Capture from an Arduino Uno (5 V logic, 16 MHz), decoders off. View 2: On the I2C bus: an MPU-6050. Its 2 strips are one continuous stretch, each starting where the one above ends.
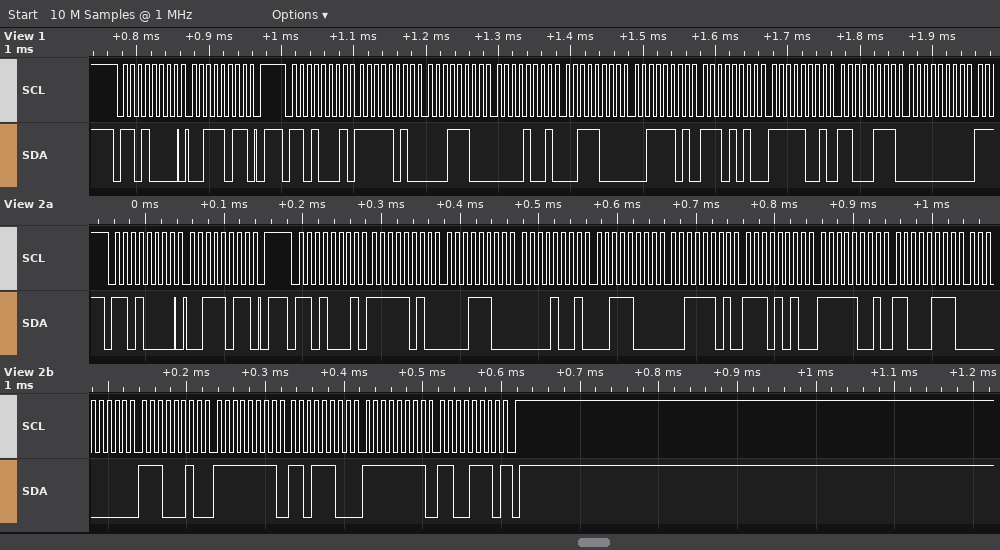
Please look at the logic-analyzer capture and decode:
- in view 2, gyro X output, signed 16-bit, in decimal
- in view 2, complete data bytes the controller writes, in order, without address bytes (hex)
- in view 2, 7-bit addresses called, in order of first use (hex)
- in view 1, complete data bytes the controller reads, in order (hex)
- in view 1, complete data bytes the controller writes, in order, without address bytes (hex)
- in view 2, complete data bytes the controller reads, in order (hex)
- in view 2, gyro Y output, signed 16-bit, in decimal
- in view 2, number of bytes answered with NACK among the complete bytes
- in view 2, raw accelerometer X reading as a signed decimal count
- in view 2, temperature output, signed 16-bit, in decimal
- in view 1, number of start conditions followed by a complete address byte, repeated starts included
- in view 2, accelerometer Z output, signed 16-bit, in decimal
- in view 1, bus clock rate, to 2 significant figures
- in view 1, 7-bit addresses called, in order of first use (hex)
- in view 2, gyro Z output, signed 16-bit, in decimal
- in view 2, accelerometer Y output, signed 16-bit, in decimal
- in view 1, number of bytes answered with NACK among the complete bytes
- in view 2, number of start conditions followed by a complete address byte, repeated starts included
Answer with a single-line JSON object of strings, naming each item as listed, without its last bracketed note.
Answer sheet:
{"in view 2, gyro X output, signed 16-bit, in decimal": "226", "in view 2, complete data bytes the controller writes, in order, without address bytes": "3B", "in view 2, 7-bit addresses called, in order of first use": "0x68", "in view 1, complete data bytes the controller reads, in order": "FA 1C 09 38 3D EA F9 C7 00", "in view 1, complete data bytes the controller writes, in order, without address bytes": "3B", "in view 2, complete data bytes the controller reads, in order": "FA 1C 09 38 3D EA F9 C7 00 E2 FF DC FF CE", "in view 2, gyro Y output, signed 16-bit, in decimal": "-36", "in view 2, number of bytes answered with NACK among the complete bytes": "1", "in view 2, raw accelerometer X reading as a signed decimal count": "-1508", "in view 2, temperature output, signed 16-bit, in decimal": "-1593", "in view 1, number of start conditions followed by a complete address byte, repeated starts included": "2", "in view 2, accelerometer Z output, signed 16-bit, in decimal": "15850", "in view 1, bus clock rate, to 2 significant figures": "100 kHz", "in view 1, 7-bit addresses called, in order of first use": "0x68", "in view 2, gyro Z output, signed 16-bit, in decimal": "-50", "in view 2, accelerometer Y output, signed 16-bit, in decimal": "2360", "in view 1, number of bytes answered with NACK among the complete bytes": "0", "in view 2, number of start conditions followed by a complete address byte, repeated starts included": "2"}
